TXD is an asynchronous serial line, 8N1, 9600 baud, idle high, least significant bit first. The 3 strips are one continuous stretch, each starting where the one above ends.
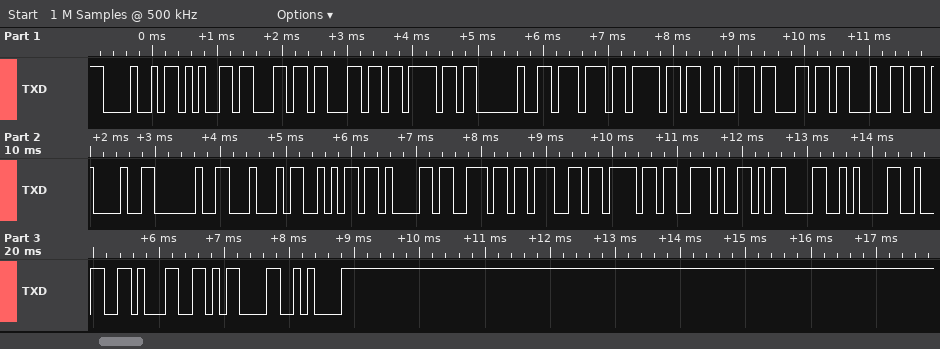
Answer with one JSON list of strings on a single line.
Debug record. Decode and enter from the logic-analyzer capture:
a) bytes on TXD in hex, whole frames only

["48 65 6C 6C 6F 20 77 6F 72 6C 64 21 20 44 6A 61 6E 67 6F 2E 0D 0A 32 31 0D 0A"]
